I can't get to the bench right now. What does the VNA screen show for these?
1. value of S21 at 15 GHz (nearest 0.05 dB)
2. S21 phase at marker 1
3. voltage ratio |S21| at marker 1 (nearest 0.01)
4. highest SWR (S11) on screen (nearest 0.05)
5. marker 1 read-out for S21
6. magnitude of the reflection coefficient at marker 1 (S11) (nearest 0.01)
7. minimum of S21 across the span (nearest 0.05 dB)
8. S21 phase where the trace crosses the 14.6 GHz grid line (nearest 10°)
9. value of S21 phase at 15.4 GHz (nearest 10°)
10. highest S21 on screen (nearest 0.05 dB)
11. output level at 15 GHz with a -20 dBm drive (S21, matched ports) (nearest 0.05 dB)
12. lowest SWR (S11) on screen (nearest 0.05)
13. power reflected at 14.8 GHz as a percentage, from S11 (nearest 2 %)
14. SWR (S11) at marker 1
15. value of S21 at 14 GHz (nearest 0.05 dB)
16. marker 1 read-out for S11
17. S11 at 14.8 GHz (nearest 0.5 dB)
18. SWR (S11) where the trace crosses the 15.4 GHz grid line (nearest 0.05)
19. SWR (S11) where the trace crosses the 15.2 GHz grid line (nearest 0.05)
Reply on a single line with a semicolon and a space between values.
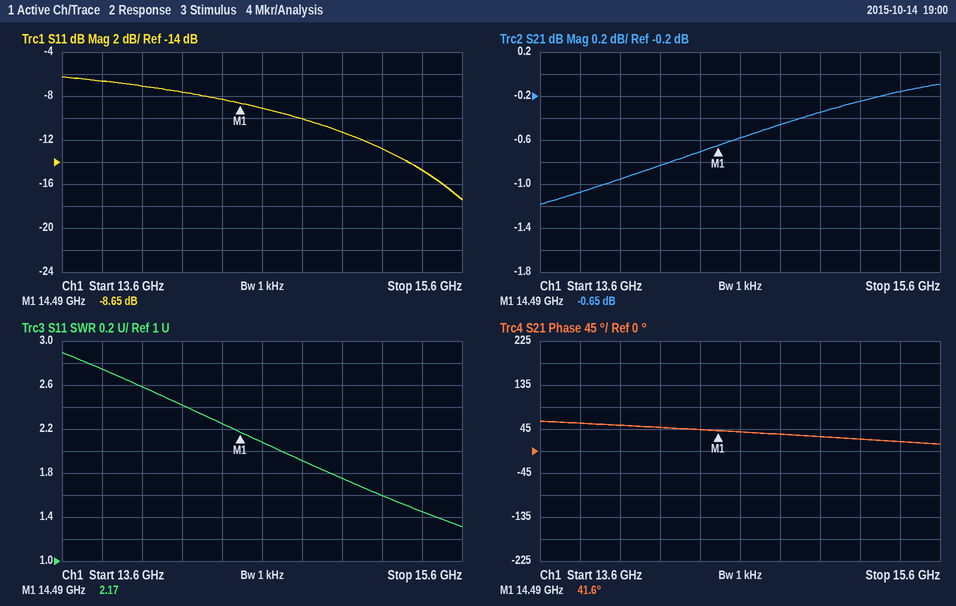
-0.35 dB; 41.6°; 0.93; 2.90; -0.65 dB; 0.37; -1.20 dB; 40°; 20°; -0.10 dB; -20.35 dBm; 1.30; 10 %; 2.17; -0.95 dB; -8.65 dB; -10.0 dB; 1.45; 1.60
